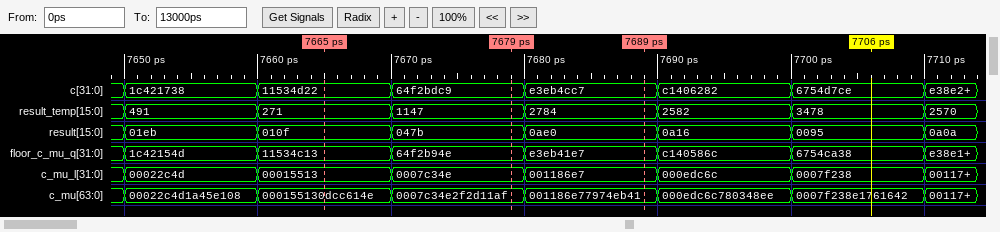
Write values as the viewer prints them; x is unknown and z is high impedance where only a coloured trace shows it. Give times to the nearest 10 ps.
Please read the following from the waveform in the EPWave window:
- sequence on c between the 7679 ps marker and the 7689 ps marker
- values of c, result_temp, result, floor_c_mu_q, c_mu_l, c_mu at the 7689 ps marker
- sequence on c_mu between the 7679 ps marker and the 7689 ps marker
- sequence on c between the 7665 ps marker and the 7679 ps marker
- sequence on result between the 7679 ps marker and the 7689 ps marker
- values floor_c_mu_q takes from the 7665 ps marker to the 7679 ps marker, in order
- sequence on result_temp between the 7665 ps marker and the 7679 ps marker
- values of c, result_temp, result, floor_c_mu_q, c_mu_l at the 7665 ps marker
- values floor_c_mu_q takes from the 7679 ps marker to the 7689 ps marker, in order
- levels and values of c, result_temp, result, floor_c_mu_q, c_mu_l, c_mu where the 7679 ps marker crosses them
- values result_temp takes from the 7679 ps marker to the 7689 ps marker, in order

64f2bdc9, e3eb4cc7
c=e3eb4cc7, result_temp=2784, result=0ae0, floor_c_mu_q=e3eb41e7, c_mu_l=001186e7, c_mu=001186e77974eb41
0007c34e2f2d11af, 001186e77974eb41
11534d22, 64f2bdc9
047b, 0ae0
11534c13, 64f2b94e
271, 1147
c=11534d22, result_temp=271, result=010f, floor_c_mu_q=11534c13, c_mu_l=00015513
64f2b94e, e3eb41e7
c=64f2bdc9, result_temp=1147, result=047b, floor_c_mu_q=64f2b94e, c_mu_l=0007c34e, c_mu=0007c34e2f2d11af
1147, 2784
